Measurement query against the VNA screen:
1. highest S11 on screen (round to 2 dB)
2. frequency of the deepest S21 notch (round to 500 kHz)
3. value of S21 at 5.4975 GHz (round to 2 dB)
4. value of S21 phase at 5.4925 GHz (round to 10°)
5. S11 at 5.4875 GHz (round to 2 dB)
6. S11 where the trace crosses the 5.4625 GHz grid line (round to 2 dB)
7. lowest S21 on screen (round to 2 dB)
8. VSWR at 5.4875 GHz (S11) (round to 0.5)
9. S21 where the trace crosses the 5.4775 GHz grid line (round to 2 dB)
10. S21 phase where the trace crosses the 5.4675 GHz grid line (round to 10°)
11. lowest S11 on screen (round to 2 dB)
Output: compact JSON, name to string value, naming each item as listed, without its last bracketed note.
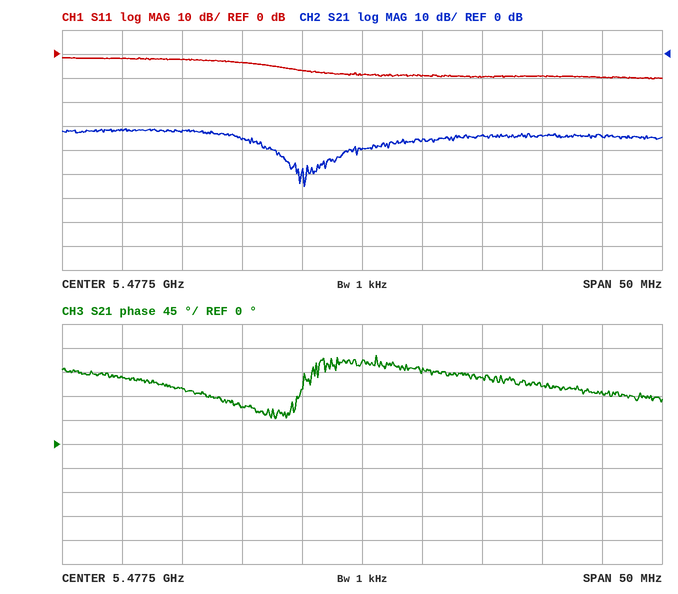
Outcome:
{"highest S11 on screen": "-2 dB", "frequency of the deepest S21 notch": "5.4725 GHz", "value of S21 at 5.4975 GHz": "-34 dB", "value of S21 phase at 5.4925 GHz": "110°", "S11 at 5.4875 GHz": "-10 dB", "S11 where the trace crosses the 5.4625 GHz grid line": "-2 dB", "lowest S21 on screen": "-56 dB", "VSWR at 5.4875 GHz (S11)": "2.0", "S21 where the trace crosses the 5.4775 GHz grid line": "-40 dB", "S21 phase where the trace crosses the 5.4675 GHz grid line": "70°", "lowest S11 on screen": "-10 dB"}
